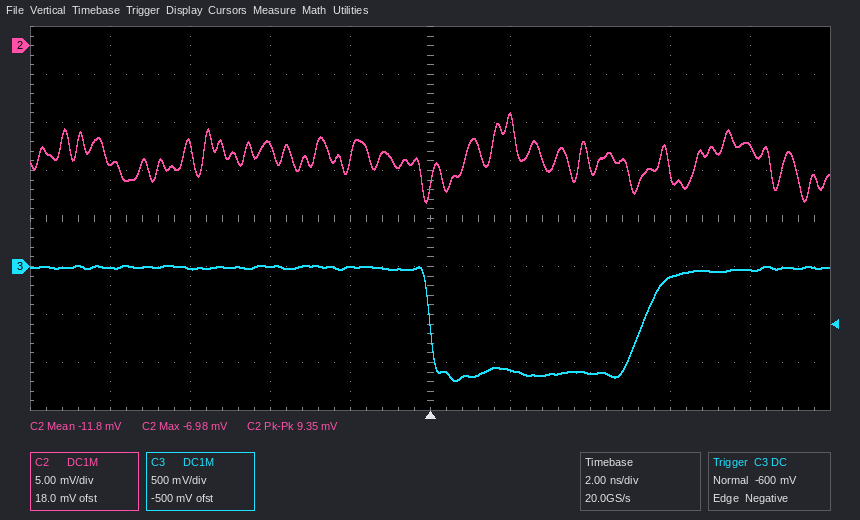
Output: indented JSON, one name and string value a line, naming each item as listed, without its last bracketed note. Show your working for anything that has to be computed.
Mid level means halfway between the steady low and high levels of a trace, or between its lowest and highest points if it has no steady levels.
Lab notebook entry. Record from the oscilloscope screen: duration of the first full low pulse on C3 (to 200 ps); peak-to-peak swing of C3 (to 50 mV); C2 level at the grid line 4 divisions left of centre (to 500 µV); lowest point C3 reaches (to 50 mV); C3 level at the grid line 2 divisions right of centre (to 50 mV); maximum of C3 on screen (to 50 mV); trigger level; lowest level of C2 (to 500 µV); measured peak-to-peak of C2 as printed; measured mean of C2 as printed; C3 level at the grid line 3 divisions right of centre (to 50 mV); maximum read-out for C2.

{
  "duration of the first full low pulse on C3": "5.4 ns",
  "peak-to-peak swing of C3": "0 mV − (-1.20 V) = 1.20 V",
  "C2 level at the grid line 4 divisions left of centre": "-12.0 mV",
  "lowest point C3 reaches": "-1.20 V",
  "C3 level at the grid line 2 divisions right of centre": "-1.10 V",
  "maximum of C3 on screen": "0 mV",
  "trigger level": "-600 mV",
  "lowest level of C2": "-16.5 mV",
  "measured peak-to-peak of C2 as printed": "9.35 mV",
  "measured mean of C2 as printed": "-11.8 mV",
  "C3 level at the grid line 3 divisions right of centre": "-100 mV",
  "maximum read-out for C2": "-6.98 mV"
}
